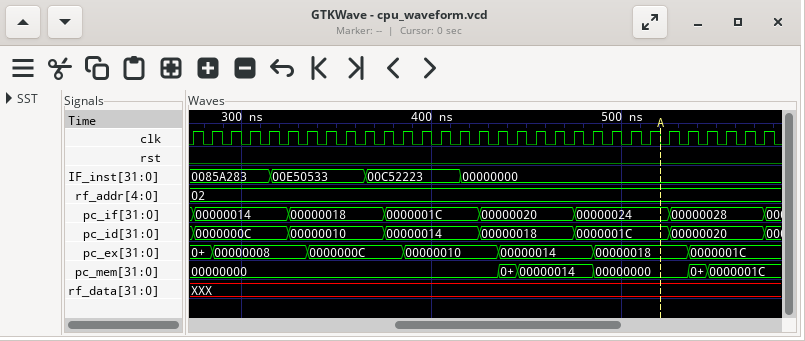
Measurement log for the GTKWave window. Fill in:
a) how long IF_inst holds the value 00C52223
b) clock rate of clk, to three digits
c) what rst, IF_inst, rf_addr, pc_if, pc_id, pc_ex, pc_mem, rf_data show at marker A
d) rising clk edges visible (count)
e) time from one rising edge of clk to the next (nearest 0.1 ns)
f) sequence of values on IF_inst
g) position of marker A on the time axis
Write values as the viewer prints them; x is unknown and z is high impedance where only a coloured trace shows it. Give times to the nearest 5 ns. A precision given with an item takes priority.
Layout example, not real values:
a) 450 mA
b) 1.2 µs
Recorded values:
a) 50 ns
b) 100 MHz
c) rst=0, IF_inst=00000000, rf_addr=02, pc_if=00000024, pc_id=0000001C, pc_ex=00000018, pc_mem=00000000, rf_data=XXX
d) 31
e) 10 ns
f) 0085A283, 00E50533, 00C52223, 00000000
g) 520 ns
